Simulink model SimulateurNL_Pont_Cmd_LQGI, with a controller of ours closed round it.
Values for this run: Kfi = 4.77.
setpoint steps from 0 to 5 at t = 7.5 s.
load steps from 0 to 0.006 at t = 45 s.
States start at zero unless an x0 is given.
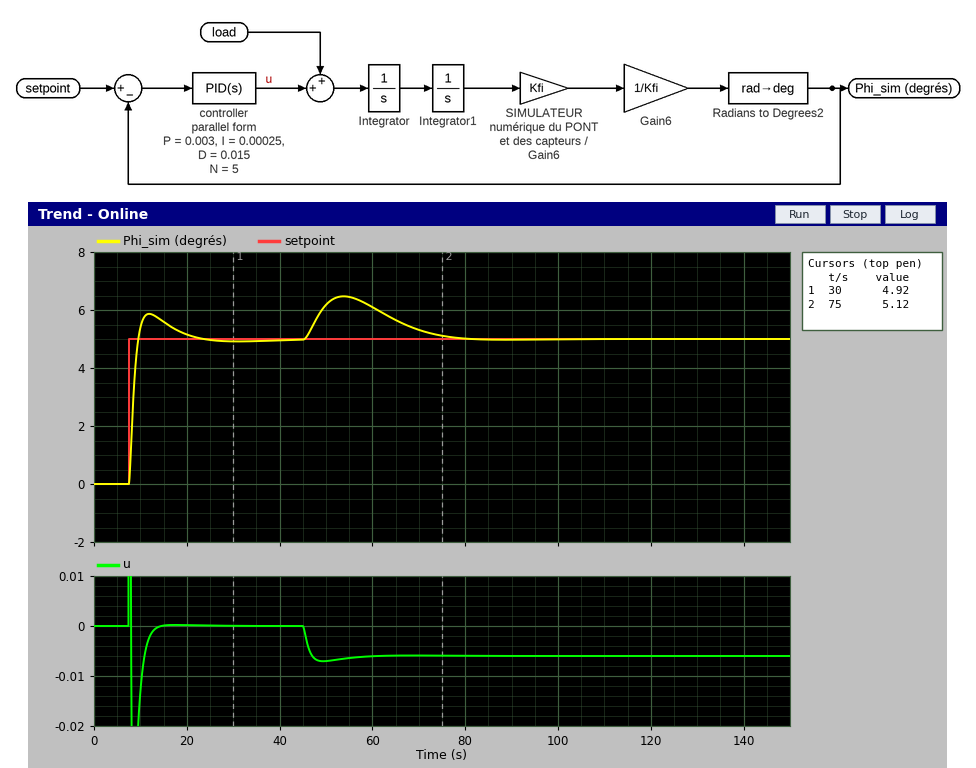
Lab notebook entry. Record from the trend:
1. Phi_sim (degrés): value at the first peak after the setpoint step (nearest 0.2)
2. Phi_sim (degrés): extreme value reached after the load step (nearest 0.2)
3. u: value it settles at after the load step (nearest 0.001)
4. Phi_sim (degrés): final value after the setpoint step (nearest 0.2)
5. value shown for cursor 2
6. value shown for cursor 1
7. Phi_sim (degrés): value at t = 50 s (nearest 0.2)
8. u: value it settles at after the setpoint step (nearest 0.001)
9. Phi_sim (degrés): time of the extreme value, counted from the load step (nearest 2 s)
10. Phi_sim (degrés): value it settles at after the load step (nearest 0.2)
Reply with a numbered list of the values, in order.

1. 5.8
2. 6.4
3. -0.006
4. 5.0
5. 5.12
6. 4.92
7. 6.2
8. 0.000
9. 8 s
10. 5.0
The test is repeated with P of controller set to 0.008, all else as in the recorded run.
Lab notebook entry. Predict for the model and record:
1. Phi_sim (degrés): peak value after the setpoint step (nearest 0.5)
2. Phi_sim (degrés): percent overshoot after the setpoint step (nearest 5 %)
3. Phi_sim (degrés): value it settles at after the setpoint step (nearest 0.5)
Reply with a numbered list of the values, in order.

1. 6.5
2. 30 %
3. 5.0
